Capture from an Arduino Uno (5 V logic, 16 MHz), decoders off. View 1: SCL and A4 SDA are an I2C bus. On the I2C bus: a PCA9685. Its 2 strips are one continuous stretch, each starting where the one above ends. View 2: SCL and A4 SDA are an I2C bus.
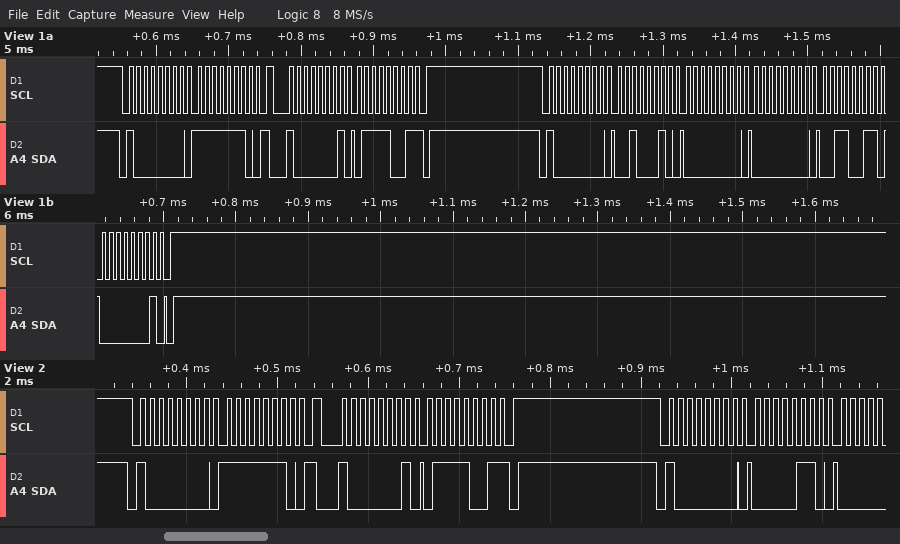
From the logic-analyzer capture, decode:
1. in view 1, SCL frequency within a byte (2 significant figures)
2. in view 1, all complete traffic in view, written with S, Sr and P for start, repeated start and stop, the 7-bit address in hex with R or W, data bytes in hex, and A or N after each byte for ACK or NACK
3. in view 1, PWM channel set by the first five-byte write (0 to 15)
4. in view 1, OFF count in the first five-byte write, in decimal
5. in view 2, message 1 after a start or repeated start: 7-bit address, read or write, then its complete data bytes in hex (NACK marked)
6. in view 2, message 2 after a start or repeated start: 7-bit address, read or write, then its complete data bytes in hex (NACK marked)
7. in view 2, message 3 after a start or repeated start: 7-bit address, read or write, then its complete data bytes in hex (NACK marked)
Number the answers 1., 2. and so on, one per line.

1. 100 kHz
2. S 40W A FE A Sr 40R A 79 N P S 40W A 22 A 00 A 00 A 33 A 01 A P
3. 7
4. 307
5. 0x40 write: FE
6. 0x40 read: 79 NACK
7. 0x40 write: 06
